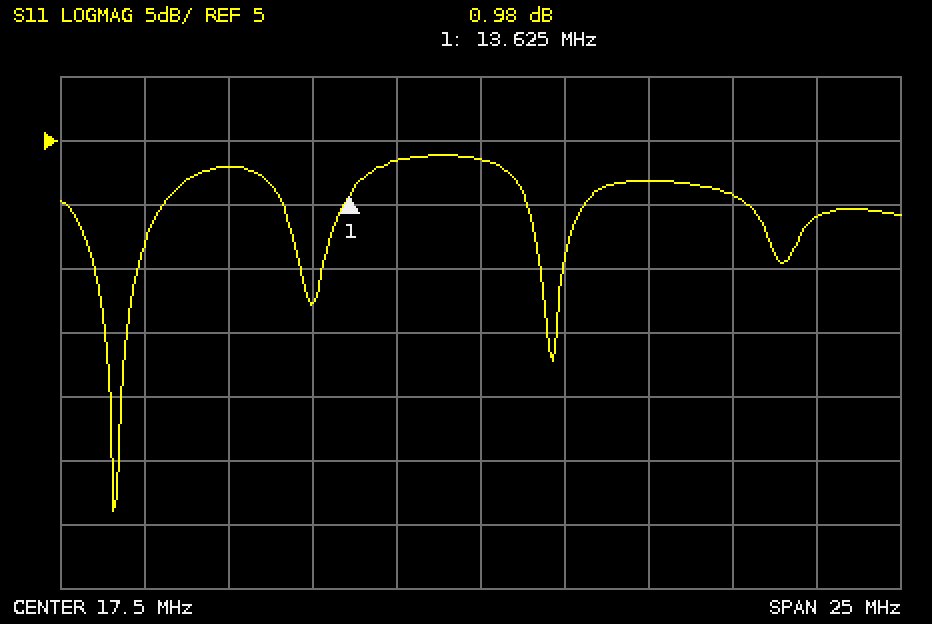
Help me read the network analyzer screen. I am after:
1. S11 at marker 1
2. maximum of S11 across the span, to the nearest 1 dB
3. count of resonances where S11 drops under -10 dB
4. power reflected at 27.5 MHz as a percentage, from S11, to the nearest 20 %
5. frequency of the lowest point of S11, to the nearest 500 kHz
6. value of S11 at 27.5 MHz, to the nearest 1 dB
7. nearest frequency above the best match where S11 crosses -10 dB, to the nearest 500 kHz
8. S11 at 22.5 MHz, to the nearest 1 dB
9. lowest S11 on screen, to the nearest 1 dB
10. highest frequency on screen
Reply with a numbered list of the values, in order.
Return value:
1. 0.98 dB
2. 4 dB
3. 2
4. 80 %
5. 6.5 MHz
6. -1 dB
7. 7.0 MHz
8. 2 dB
9. -24 dB
10. 30 MHz
